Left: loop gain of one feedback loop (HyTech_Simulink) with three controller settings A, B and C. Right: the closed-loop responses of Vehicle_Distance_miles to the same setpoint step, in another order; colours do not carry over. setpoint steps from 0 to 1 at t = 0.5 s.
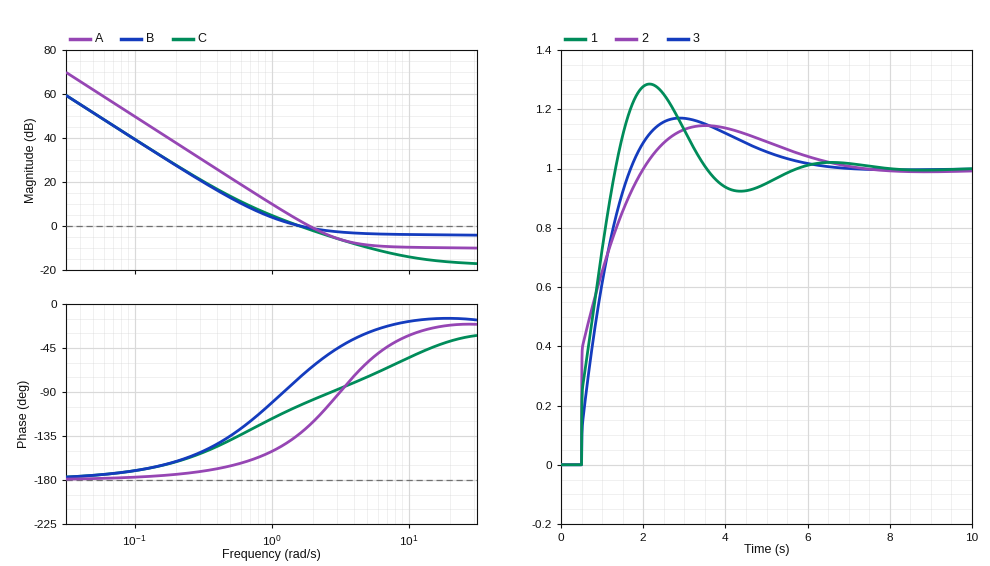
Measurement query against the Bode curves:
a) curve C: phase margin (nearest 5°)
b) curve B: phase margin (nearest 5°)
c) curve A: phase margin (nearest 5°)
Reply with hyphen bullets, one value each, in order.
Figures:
- 75°
- 105°
- 55°
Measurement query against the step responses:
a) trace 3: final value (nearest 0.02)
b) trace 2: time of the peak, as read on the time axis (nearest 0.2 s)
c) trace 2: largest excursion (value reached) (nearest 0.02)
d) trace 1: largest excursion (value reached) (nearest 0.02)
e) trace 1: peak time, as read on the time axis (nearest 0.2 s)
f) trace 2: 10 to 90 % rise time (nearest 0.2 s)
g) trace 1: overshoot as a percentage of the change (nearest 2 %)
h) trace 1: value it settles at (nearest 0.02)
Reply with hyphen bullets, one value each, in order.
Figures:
- 1.00
- 3.6 s
- 1.14
- 1.28
- 2.2 s
- 1.2 s
- 28 %
- 1.00
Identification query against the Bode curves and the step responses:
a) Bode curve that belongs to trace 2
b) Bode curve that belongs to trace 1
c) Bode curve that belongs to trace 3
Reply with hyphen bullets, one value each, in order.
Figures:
- B
- A
- C
